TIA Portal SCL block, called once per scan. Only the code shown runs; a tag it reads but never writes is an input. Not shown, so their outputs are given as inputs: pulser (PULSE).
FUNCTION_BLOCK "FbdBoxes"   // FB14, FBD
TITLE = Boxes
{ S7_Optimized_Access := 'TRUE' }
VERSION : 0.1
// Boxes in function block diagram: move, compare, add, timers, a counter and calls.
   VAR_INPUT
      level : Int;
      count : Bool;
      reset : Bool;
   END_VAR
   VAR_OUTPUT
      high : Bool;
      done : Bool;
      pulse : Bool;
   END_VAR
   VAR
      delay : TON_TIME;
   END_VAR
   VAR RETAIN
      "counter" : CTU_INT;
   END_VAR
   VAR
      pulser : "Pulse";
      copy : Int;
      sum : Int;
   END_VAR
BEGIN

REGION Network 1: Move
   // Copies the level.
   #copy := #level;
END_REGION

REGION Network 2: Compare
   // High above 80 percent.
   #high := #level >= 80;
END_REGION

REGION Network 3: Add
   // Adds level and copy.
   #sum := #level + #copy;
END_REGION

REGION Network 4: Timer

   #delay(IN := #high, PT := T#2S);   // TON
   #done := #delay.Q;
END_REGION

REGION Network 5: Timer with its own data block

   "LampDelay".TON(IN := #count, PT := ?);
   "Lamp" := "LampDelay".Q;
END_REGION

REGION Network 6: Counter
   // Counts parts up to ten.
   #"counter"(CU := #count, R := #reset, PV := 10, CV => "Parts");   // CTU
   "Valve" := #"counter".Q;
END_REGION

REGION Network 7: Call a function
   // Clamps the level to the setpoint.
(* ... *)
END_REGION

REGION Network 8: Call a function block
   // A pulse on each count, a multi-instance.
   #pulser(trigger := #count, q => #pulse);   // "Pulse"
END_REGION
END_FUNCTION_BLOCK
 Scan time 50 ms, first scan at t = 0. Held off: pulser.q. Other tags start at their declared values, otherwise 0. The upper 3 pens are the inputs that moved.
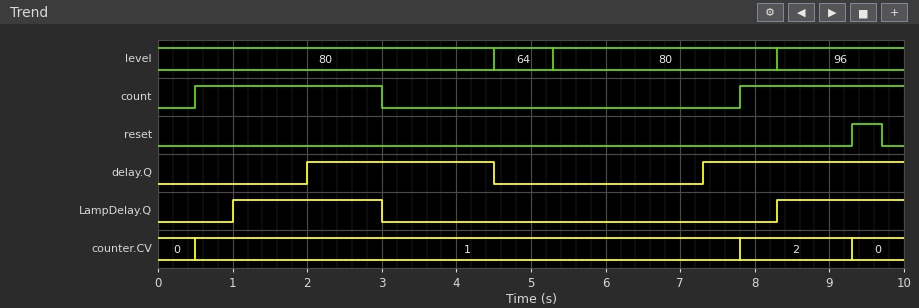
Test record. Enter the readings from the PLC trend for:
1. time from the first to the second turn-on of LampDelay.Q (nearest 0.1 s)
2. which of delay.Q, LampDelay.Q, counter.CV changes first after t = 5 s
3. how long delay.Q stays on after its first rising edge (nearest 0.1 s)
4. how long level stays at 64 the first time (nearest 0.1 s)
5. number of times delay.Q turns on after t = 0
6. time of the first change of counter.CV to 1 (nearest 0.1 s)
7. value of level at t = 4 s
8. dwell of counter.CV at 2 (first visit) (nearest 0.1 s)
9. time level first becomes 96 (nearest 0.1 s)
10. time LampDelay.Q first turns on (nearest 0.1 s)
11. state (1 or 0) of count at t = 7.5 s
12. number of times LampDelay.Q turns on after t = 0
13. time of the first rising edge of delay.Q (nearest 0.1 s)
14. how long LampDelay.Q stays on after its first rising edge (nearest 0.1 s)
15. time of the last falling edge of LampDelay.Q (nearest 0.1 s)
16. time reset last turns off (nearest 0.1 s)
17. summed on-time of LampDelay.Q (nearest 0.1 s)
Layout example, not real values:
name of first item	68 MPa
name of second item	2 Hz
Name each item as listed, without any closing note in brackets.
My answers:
time from the first to the second turn-on of LampDelay.Q	7.3 s
which of delay.Q, LampDelay.Q, counter.CV changes first after t = 5 s	delay.Q
how long delay.Q stays on after its first rising edge	2.5 s
how long level stays at 64 the first time	0.8 s
number of times delay.Q turns on after t = 0	2
time of the first change of counter.CV to 1	0.5 s
value of level at t = 4 s	80
dwell of counter.CV at 2 (first visit)	1.5 s
time level first becomes 96	8.3 s
time LampDelay.Q first turns on	1.0 s
state (1 or 0) of count at t = 7.5 s	0
number of times LampDelay.Q turns on after t = 0	2
time of the first rising edge of delay.Q	2.0 s
how long LampDelay.Q stays on after its first rising edge	2.0 s
time of the last falling edge of LampDelay.Q	3.0 s
time reset last turns off	9.7 s
summed on-time of LampDelay.Q	3.7 s
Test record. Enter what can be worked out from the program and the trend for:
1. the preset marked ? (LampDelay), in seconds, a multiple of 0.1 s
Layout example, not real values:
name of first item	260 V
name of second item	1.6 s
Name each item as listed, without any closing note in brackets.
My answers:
the preset marked ? (LampDelay), in seconds, a multiple of 0.1 s	0.5 s
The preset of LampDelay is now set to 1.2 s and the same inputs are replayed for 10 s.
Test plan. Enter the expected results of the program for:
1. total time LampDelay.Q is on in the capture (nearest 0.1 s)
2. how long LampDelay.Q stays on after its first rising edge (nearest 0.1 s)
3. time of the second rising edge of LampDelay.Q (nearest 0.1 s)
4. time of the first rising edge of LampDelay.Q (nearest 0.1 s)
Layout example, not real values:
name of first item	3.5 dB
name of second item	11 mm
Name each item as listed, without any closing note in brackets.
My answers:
total time LampDelay.Q is on in the capture	2.3 s
how long LampDelay.Q stays on after its first rising edge	1.3 s
time of the second rising edge of LampDelay.Q	9.0 s
time of the first rising edge of LampDelay.Q	1.7 s
